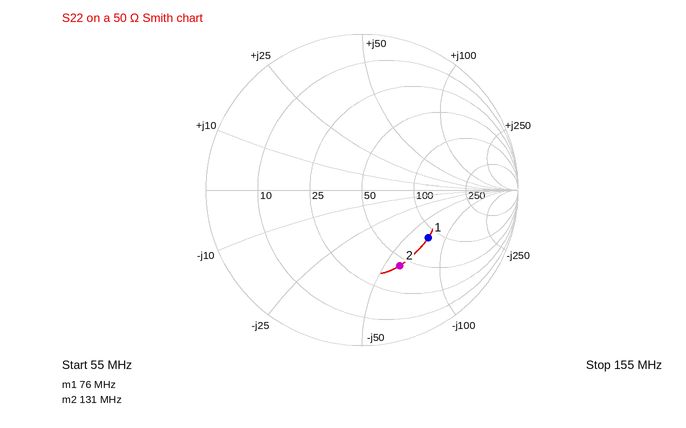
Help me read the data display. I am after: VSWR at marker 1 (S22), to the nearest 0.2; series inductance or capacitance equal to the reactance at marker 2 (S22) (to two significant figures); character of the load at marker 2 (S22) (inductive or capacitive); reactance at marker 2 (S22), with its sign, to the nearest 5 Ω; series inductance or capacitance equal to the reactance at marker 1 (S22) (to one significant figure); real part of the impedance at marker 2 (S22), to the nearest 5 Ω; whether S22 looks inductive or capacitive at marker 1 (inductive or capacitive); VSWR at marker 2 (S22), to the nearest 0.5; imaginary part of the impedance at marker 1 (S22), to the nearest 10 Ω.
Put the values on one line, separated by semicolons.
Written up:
3.2; 20 pF; capacitive; -60 Ω; 30 pF; 45 Ω; capacitive; 3.5; -70 Ω
